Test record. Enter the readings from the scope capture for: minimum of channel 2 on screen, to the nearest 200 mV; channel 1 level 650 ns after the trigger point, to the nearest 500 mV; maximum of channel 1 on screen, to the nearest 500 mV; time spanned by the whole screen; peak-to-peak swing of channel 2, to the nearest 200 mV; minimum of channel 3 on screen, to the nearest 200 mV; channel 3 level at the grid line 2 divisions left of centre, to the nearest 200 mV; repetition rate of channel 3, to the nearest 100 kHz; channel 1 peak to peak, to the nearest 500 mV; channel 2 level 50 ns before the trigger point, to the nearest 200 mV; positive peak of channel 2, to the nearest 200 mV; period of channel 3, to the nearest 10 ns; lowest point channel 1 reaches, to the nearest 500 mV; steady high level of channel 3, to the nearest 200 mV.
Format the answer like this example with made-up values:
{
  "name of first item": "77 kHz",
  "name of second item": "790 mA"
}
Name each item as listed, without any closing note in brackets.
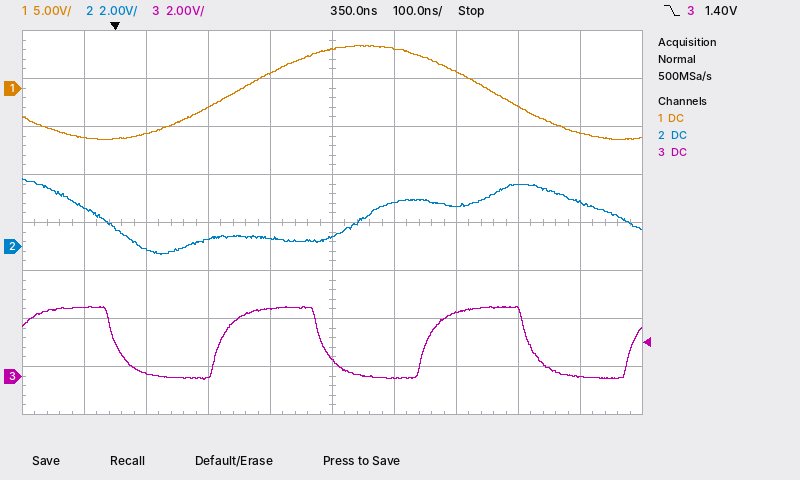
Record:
{
  "minimum of channel 2 on screen, to the nearest 200 mV": "-400 mV",
  "channel 1 level 650 ns after the trigger point, to the nearest 500 mV": "-2.0 V",
  "maximum of channel 1 on screen, to the nearest 500 mV": "4.5 V",
  "time spanned by the whole screen": "1 µs",
  "peak-to-peak swing of channel 2, to the nearest 200 mV": "3.2 V",
  "minimum of channel 3 on screen, to the nearest 200 mV": "-200 mV",
  "channel 3 level at the grid line 2 divisions left of centre, to the nearest 200 mV": "0.0 V",
  "repetition rate of channel 3, to the nearest 100 kHz": "3.0 MHz",
  "channel 1 peak to peak, to the nearest 500 mV": "10.0 V",
  "channel 2 level 50 ns before the trigger point, to the nearest 200 mV": "1.6 V",
  "positive peak of channel 2, to the nearest 200 mV": "2.8 V",
  "period of channel 3, to the nearest 10 ns": "330 ns",
  "lowest point channel 1 reaches, to the nearest 500 mV": "-5.5 V",
  "steady high level of channel 3, to the nearest 200 mV": "2.8 V"
}
